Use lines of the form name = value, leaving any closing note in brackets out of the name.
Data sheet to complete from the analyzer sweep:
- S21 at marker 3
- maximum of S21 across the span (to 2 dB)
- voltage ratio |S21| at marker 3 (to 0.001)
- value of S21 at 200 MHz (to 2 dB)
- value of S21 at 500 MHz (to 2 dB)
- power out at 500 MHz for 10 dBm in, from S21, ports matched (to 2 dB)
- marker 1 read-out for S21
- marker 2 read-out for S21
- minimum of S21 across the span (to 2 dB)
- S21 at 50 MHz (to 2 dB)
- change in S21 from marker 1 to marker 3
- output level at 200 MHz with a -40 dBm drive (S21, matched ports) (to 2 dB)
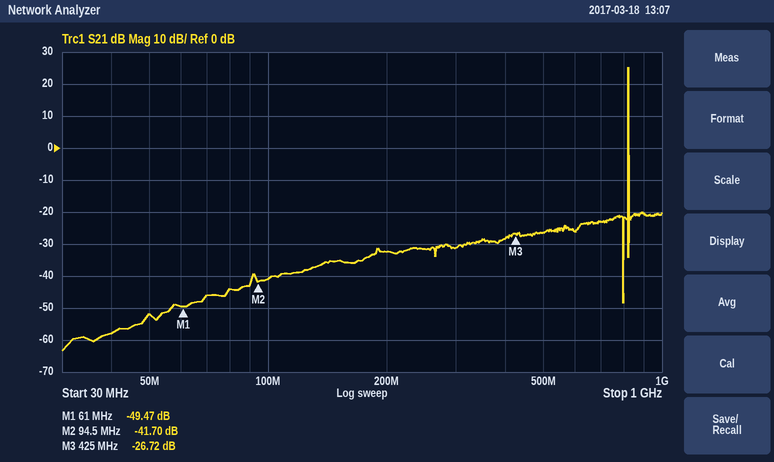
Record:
S21 at marker 3 = -26.72 dB
maximum of S21 across the span = 26 dB
voltage ratio |S21| at marker 3 = 0.046
value of S21 at 200 MHz = -32 dB
value of S21 at 500 MHz = -26 dB
power out at 500 MHz for 10 dBm in, from S21, ports matched = -16 dBm
marker 1 read-out for S21 = -49.47 dB
marker 2 read-out for S21 = -41.70 dB
minimum of S21 across the span = -64 dB
S21 at 50 MHz = -52 dB
change in S21 from marker 1 to marker 3 = 22.75 dB
output level at 200 MHz with a -40 dBm drive (S21, matched ports) = -72 dBm
